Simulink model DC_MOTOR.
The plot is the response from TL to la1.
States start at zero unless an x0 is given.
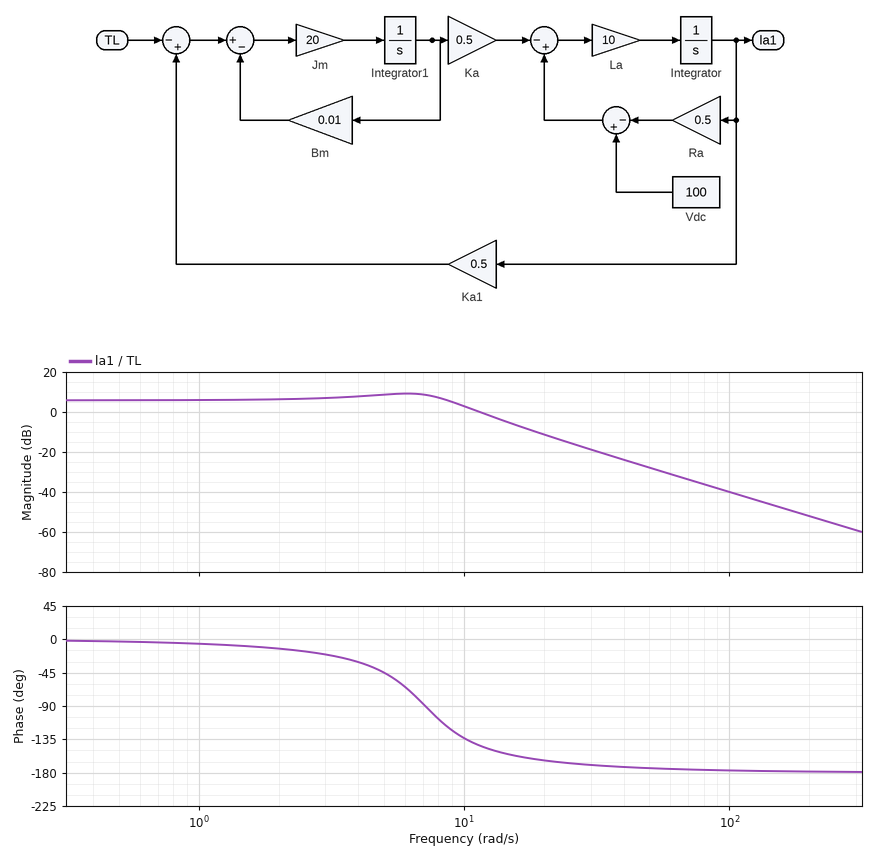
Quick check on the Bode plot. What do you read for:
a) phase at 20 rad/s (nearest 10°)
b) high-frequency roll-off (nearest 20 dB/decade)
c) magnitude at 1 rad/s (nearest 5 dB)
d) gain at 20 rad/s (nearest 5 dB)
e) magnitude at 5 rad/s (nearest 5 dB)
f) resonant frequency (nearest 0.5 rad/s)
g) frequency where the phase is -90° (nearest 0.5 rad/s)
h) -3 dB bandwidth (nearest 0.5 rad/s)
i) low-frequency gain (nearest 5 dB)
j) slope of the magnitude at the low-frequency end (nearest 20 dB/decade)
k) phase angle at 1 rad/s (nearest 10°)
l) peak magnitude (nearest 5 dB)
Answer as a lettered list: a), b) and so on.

a) -160°
b) -40 dB/decade
c) 5 dB
d) -10 dB
e) 10 dB
f) 6.0 rad/s
g) 7.0 rad/s
h) 10.0 rad/s
i) 5 dB
j) 0 dB/decade
k) -10°
l) 10 dB
